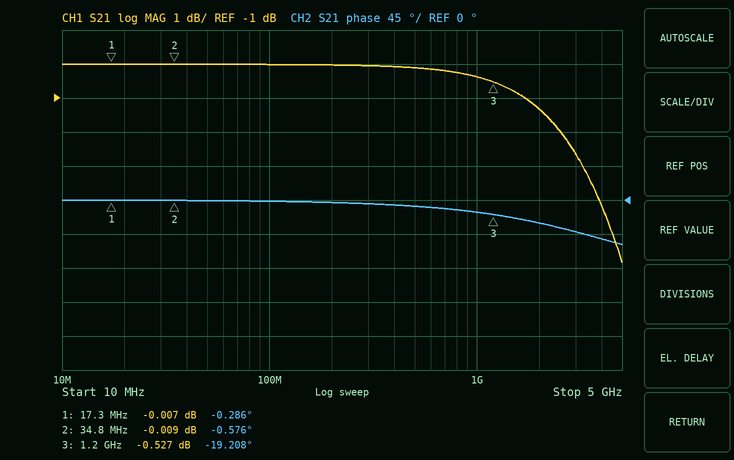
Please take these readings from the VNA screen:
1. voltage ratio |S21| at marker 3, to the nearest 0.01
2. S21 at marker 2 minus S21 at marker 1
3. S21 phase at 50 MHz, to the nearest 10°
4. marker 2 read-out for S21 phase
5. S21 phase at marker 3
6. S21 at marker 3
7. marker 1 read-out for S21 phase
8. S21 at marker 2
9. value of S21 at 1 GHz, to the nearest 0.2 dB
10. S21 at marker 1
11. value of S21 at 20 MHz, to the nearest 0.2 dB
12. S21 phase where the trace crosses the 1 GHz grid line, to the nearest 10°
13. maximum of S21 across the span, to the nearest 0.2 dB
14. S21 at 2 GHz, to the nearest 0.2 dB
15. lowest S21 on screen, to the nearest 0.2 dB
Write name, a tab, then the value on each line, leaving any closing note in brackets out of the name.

voltage ratio |S21| at marker 3, to the nearest 0.01	0.94
S21 at marker 2 minus S21 at marker 1	-0.002 dB
S21 phase at 50 MHz, to the nearest 10°	0°
marker 2 read-out for S21 phase	-0.576°
S21 phase at marker 3	-19.208°
S21 at marker 3	-0.527 dB
marker 1 read-out for S21 phase	-0.286°
S21 at marker 2	-0.009 dB
value of S21 at 1 GHz, to the nearest 0.2 dB	-0.4 dB
S21 at marker 1	-0.007 dB
value of S21 at 20 MHz, to the nearest 0.2 dB	0.0 dB
S21 phase where the trace crosses the 1 GHz grid line, to the nearest 10°	-20°
maximum of S21 across the span, to the nearest 0.2 dB	0.0 dB
S21 at 2 GHz, to the nearest 0.2 dB	-1.4 dB
lowest S21 on screen, to the nearest 0.2 dB	-5.8 dB
